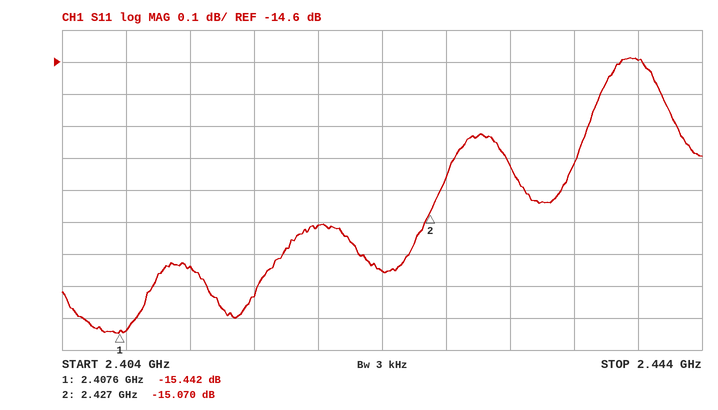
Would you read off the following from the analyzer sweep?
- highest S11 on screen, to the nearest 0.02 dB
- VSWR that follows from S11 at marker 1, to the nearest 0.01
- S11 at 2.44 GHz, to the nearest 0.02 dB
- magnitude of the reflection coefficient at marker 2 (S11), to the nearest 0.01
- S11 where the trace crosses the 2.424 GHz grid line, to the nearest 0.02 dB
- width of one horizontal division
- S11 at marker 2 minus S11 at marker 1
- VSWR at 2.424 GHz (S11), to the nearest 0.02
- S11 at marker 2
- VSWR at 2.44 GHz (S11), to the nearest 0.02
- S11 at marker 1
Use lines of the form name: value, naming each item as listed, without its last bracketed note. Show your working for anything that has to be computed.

highest S11 on screen, to the nearest 0.02 dB: -14.58 dB
VSWR that follows from S11 at marker 1, to the nearest 0.01: (1 + 0.1690)/(1 − 0.1690) ≈ 1.41
S11 at 2.44 GHz, to the nearest 0.02 dB: -14.60 dB
magnitude of the reflection coefficient at marker 2 (S11), to the nearest 0.01: 10^(-15.07/20) ≈ 0.18
S11 where the trace crosses the 2.424 GHz grid line, to the nearest 0.02 dB: -15.26 dB
width of one horizontal division: 4 MHz
S11 at marker 2 minus S11 at marker 1: -15.07 − (-15.442) = 0.372 dB
VSWR at 2.424 GHz (S11), to the nearest 0.02: |Γ| = 10^(-15.26/20) = 0.1726; VSWR = (1 + 0.1726)/(1 − 0.1726) ≈ 1.42
S11 at marker 2: -15.070 dB
VSWR at 2.44 GHz (S11), to the nearest 0.02: |Γ| = 10^(-14.6/20) = 0.1862; VSWR = (1 + 0.1862)/(1 − 0.1862) ≈ 1.46
S11 at marker 1: -15.442 dB
